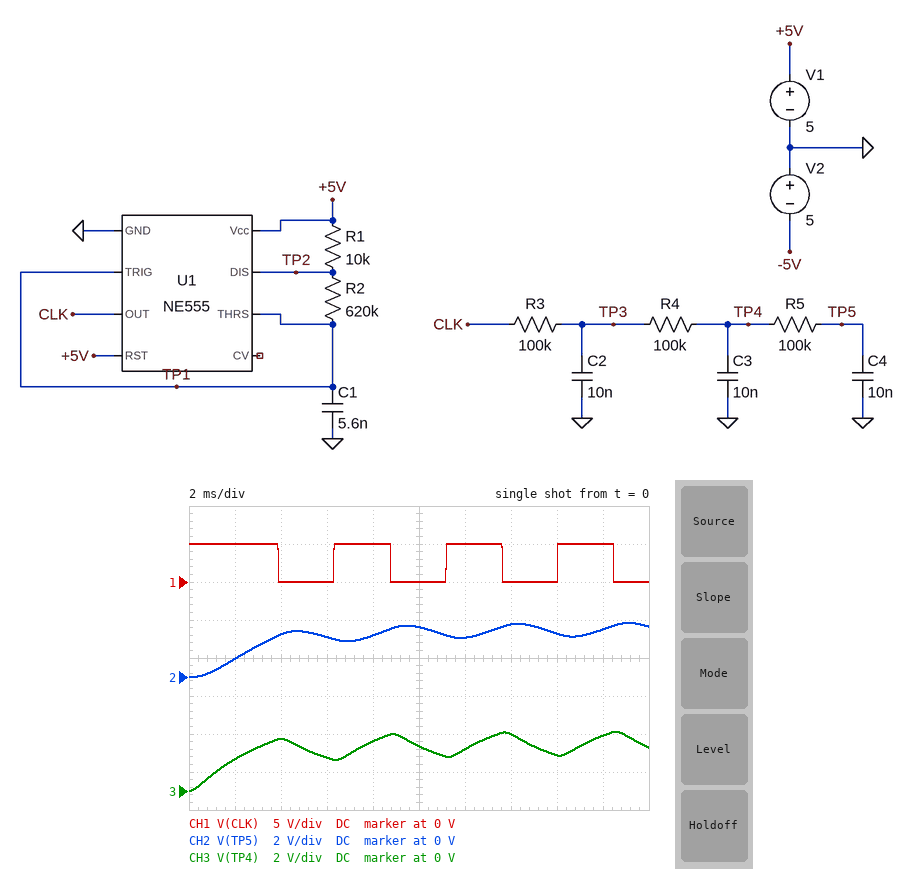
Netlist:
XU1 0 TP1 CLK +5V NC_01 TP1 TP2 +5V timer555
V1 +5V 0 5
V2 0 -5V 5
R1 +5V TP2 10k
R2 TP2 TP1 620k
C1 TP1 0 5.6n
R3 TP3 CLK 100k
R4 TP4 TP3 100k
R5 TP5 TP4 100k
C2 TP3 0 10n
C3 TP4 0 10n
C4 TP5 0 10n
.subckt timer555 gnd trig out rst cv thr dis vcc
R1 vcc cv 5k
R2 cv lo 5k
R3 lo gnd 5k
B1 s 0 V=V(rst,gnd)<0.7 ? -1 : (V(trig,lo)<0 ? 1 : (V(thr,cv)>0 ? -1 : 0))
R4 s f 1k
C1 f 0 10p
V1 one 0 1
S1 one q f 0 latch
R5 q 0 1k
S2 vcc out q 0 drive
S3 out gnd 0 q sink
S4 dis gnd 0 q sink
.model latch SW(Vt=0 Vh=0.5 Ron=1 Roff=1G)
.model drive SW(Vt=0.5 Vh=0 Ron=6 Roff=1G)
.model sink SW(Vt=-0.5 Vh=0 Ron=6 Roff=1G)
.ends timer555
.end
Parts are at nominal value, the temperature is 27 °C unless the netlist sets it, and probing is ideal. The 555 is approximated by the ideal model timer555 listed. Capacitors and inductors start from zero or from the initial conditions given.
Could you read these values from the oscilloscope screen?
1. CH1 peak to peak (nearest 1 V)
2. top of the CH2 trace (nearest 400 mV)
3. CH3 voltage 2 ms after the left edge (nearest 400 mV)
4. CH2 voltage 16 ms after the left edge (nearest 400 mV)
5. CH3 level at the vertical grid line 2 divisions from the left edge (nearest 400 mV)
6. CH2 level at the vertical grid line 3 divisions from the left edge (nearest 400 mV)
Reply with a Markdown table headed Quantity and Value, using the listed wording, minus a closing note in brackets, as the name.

| Quantity | Value |
|---|---|
| CH1 peak to peak | 5 V |
| top of the CH2 trace | 2.8 V |
| CH3 voltage 2 ms after the left edge | 1.6 V |
| CH2 voltage 16 ms after the left edge | 2.4 V |
| CH3 level at the vertical grid line 2 divisions from the left edge | 2.8 V |
| CH2 level at the vertical grid line 3 divisions from the left edge | 2.0 V |
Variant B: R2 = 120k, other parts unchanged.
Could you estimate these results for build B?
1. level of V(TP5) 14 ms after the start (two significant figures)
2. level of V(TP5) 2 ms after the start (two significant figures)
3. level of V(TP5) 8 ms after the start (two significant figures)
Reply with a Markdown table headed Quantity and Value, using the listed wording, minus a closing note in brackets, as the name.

| Quantity | Value |
|---|---|
| level of V(TP5) 14 ms after the start | 2.4 V |
| level of V(TP5) 2 ms after the start | 690 mV |
| level of V(TP5) 8 ms after the start | 2.0 V |
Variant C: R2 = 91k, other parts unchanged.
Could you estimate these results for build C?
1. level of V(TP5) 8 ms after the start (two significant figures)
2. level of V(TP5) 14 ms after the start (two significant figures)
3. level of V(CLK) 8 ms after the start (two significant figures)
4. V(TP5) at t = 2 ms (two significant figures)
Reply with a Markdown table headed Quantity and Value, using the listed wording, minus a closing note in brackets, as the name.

| Quantity | Value |
|---|---|
| level of V(TP5) 8 ms after the start | 2.0 V |
| level of V(TP5) 14 ms after the start | 2.4 V |
| level of V(CLK) 8 ms after the start | 5.0 V |
| V(TP5) at t = 2 ms | 640 mV |
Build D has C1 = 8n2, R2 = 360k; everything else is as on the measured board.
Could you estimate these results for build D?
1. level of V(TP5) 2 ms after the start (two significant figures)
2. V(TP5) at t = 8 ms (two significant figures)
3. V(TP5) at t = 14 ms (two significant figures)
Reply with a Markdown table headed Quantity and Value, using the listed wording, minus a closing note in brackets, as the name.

| Quantity | Value |
|---|---|
| level of V(TP5) 2 ms after the start | 960 mV |
| V(TP5) at t = 8 ms | 2.5 V |
| V(TP5) at t = 14 ms | 2.2 V |
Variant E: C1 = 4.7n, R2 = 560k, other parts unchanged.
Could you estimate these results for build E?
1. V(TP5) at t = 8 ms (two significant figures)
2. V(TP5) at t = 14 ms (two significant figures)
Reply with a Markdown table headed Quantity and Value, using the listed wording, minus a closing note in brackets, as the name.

| Quantity | Value |
|---|---|
| V(TP5) at t = 8 ms | 2.3 V |
| V(TP5) at t = 14 ms | 2.5 V |
